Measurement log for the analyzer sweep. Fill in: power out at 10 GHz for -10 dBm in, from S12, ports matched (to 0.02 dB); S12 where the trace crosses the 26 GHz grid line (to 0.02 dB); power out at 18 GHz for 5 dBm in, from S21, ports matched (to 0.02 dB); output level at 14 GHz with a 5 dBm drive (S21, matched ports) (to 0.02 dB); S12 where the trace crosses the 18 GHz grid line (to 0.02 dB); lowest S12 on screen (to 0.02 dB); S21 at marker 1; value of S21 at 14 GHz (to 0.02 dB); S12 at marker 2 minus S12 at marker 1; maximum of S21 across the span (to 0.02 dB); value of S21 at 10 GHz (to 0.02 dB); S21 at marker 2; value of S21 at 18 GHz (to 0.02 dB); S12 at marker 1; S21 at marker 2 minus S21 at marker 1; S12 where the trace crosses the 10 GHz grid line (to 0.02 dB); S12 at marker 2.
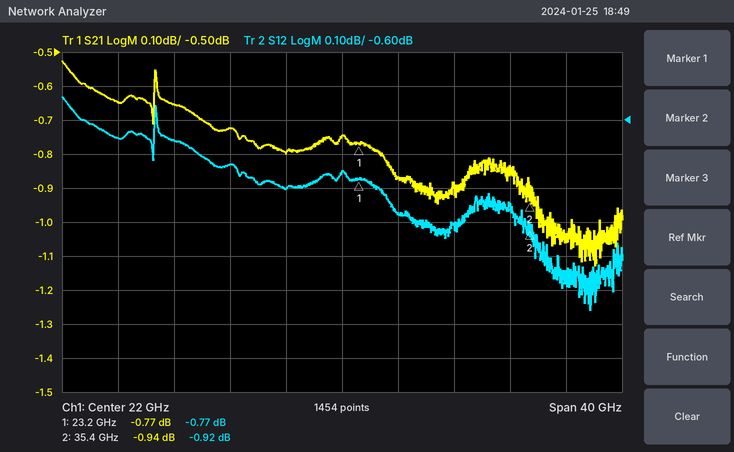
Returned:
-10.66 dBm
-0.88 dB
4.20 dBm
4.28 dBm
-0.80 dB
-1.16 dB
-0.77 dB
-0.72 dB
-0.15 dB
-0.52 dB
-0.66 dB
-0.94 dB
-0.80 dB
-0.77 dB
-0.17 dB
-0.66 dB
-0.92 dB
